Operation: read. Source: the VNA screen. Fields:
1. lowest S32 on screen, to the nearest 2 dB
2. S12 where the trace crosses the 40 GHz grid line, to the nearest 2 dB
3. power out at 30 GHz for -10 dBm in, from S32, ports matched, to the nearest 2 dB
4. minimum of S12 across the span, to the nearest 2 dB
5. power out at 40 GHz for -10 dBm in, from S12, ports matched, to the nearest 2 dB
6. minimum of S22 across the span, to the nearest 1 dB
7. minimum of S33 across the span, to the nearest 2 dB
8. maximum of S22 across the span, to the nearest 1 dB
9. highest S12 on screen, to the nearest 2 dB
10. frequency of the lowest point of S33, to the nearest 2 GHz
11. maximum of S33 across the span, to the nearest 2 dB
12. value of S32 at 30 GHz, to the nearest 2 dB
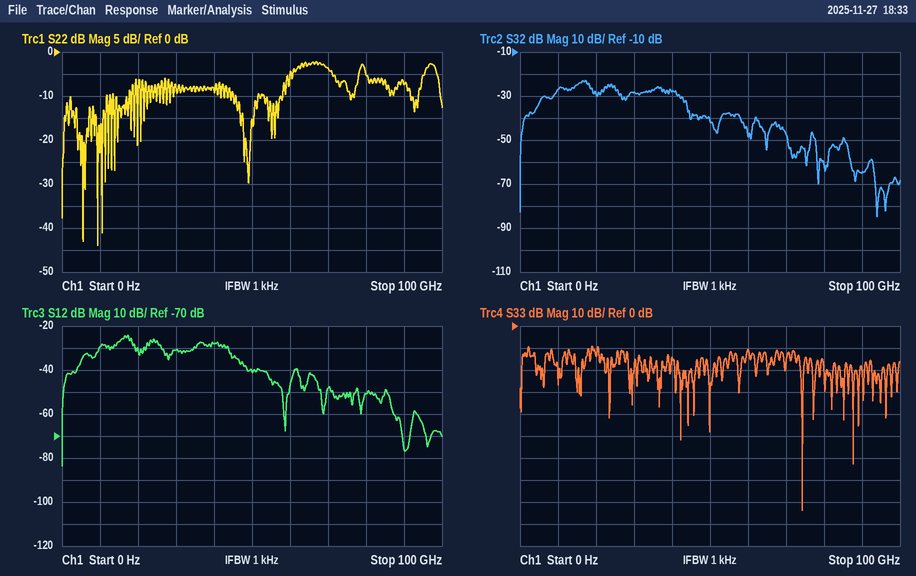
-84 dB
-28 dB
-38 dBm
-84 dB
-38 dBm
-44 dB
-84 dB
-2 dB
-24 dB
74 GHz
-10 dB
-28 dB
